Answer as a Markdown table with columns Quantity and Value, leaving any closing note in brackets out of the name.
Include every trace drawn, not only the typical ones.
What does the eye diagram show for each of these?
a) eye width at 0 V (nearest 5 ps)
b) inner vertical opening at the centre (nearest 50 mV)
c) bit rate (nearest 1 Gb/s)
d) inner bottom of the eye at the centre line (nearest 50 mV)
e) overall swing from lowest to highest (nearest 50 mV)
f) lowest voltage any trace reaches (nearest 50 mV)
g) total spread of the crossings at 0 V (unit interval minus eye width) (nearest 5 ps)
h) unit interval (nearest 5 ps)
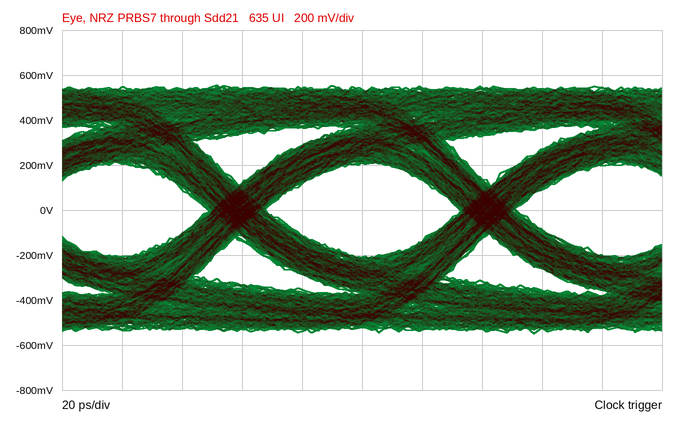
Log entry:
| Quantity | Value |
|---|---|
| eye width at 0 V | 65 ps |
| inner vertical opening at the centre | 400 mV |
| bit rate | 12 Gb/s |
| inner bottom of the eye at the centre line | -200 mV |
| overall swing from lowest to highest | 1.10 V |
| lowest voltage any trace reaches | -550 mV |
| total spread of the crossings at 0 V (unit interval minus eye width) | 20 ps |
| unit interval | 85 ps |
